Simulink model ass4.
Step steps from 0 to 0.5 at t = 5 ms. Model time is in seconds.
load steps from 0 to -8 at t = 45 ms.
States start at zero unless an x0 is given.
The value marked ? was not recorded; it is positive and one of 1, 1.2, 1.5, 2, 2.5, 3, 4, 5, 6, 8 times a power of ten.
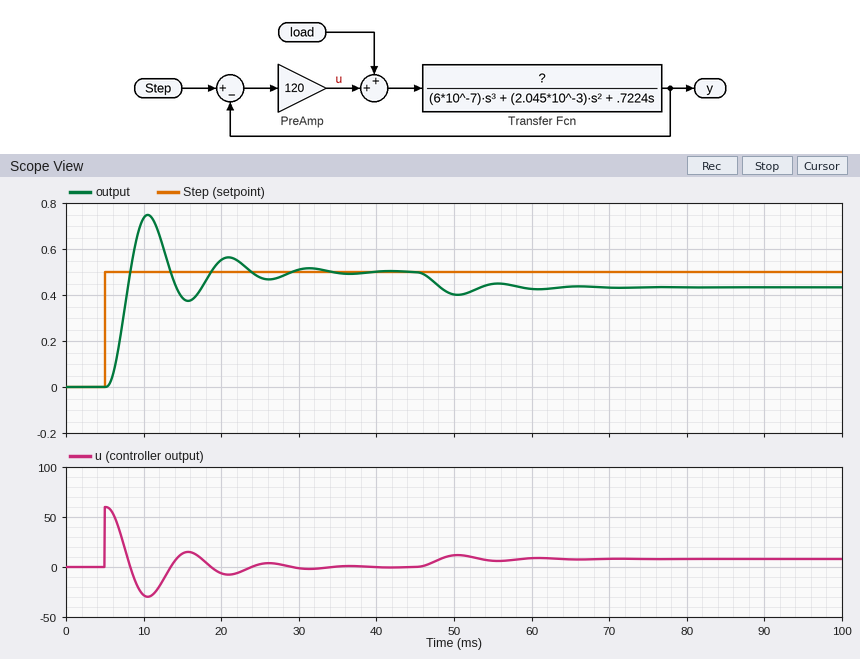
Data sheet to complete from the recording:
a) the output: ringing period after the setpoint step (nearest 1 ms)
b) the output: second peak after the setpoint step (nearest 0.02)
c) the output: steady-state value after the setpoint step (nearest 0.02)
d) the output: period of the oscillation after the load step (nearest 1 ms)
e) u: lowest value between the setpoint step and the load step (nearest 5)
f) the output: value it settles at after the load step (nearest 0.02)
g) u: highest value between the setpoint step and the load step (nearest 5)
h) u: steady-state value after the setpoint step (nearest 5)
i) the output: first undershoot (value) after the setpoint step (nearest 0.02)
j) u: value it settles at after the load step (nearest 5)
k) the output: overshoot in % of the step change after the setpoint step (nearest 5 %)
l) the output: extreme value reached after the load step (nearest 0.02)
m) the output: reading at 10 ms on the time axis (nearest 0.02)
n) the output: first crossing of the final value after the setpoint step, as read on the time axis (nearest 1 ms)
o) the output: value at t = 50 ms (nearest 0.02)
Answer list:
10 ms
0.56
0.50
10 ms
-30
0.44
60
0
0.38
10
50 %
0.40
0.74
8 ms
0.40
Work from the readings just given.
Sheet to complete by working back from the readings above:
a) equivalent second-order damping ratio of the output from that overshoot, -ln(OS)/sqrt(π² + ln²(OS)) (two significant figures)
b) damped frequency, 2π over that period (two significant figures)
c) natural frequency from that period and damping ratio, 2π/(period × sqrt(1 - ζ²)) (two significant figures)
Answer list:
0.22
0.63 rad/ms
0.64 rad/ms
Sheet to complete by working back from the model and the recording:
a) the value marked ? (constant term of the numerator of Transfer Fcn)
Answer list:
6
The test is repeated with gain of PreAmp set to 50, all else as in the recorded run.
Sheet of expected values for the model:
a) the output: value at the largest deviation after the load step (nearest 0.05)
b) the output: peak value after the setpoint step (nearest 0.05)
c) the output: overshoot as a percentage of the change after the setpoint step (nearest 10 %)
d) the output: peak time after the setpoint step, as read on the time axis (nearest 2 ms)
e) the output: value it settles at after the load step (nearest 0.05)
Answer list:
0.30
0.60
20 %
14 ms
0.35
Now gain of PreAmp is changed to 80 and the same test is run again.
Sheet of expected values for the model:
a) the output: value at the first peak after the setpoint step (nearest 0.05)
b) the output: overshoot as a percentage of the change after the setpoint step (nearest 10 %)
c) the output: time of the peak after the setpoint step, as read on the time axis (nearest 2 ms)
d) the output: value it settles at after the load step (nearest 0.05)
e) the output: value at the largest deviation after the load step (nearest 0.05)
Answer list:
0.70
40 %
12 ms
0.40
0.35
